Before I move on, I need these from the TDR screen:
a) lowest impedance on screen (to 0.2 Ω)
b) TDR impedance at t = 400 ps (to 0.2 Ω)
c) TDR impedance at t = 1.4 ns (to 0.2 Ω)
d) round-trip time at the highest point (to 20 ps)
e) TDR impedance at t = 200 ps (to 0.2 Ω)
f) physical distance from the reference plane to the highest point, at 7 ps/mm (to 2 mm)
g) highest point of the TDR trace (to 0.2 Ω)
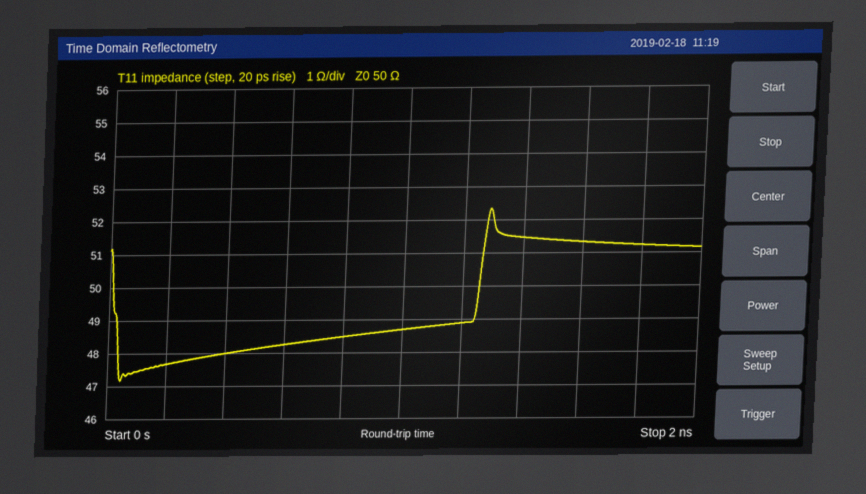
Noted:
47.2 Ω
48.0 Ω
51.4 Ω
1.28 ns
47.6 Ω
92 mm
52.4 Ω
